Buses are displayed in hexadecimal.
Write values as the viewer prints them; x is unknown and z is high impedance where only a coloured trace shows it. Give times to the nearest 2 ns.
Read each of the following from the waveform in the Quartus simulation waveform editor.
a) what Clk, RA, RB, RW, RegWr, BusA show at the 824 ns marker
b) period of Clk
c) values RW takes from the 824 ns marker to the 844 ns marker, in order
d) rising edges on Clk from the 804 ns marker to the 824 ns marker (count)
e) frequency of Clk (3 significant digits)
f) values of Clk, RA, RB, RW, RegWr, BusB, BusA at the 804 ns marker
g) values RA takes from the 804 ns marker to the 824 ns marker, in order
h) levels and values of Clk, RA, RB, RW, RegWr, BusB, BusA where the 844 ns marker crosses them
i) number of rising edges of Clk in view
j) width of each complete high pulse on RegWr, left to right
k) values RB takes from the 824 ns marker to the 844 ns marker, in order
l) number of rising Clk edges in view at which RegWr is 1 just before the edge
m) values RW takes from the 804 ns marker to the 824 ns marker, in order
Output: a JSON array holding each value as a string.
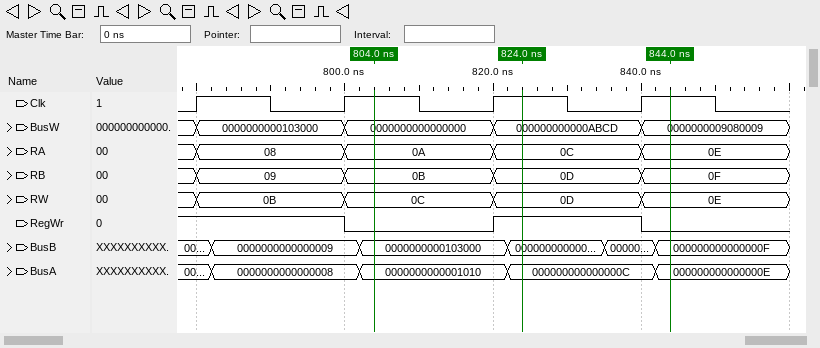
["Clk=1, RA=0C, RB=0D, RW=0D, RegWr=1, BusA=000000000000000C", "20 ns", "0D, 0E", "1", "50.0 MHz", "Clk=1, RA=0A, RB=0B, RW=0C, RegWr=0, BusB=0000000000103000, BusA=0000000000001010", "0A, 0C", "Clk=1, RA=0E, RB=0F, RW=0E, RegWr=0, BusB=000000000000000F, BusA=000000000000000E", "4", "20 ns", "0D, 0F", "3", "0C, 0D"]
